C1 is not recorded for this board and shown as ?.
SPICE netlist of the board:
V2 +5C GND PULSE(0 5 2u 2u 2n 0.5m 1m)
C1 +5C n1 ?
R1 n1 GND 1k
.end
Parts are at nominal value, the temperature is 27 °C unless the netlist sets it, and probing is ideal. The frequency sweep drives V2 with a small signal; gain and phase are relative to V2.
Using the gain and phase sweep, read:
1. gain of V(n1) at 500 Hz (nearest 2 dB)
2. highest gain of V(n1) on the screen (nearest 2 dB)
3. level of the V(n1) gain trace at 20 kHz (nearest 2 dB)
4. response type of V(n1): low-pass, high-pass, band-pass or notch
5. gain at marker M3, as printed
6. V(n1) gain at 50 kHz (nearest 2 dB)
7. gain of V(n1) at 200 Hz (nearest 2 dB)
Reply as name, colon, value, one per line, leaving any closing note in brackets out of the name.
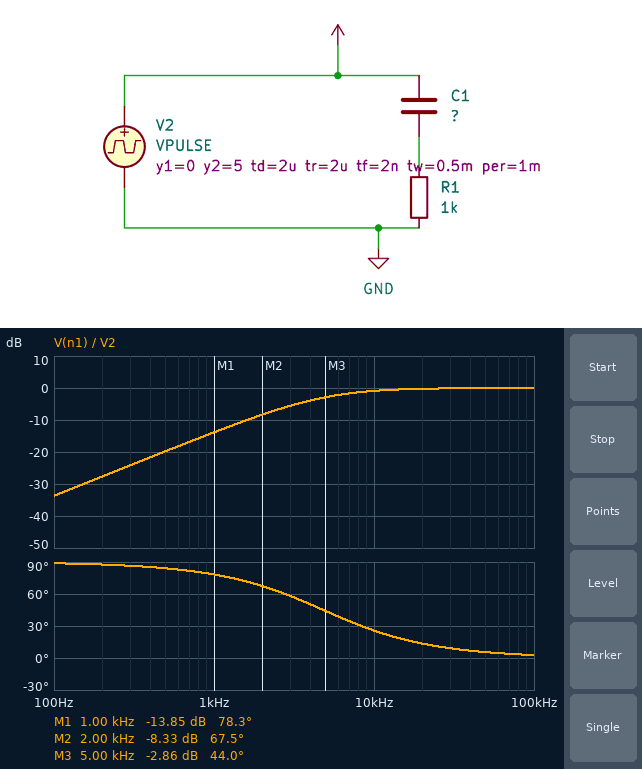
gain of V(n1) at 500 Hz: -20 dB
highest gain of V(n1) on the screen: 0 dB
level of the V(n1) gain trace at 20 kHz: 0 dB
response type of V(n1): low-pass, high-pass, band-pass or notch: high-pass
gain at marker M3, as printed: -2.86 dB
V(n1) gain at 50 kHz: 0 dB
gain of V(n1) at 200 Hz: -28 dB
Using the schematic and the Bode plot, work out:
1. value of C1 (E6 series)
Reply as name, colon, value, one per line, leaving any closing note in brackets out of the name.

value of C1: 33 nF
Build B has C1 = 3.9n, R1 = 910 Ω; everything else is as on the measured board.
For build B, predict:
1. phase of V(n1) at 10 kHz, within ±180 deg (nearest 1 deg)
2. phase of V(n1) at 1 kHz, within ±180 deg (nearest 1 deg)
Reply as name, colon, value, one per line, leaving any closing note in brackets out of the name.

phase of V(n1) at 10 kHz, within ±180 deg: 77 deg
phase of V(n1) at 1 kHz, within ±180 deg: 89 deg
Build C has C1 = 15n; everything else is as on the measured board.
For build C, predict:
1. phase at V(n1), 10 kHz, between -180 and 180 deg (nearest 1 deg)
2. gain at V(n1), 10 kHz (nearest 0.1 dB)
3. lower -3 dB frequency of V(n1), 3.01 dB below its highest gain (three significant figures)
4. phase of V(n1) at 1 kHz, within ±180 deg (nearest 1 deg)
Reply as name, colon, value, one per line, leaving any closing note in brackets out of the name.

phase at V(n1), 10 kHz, between -180 and 180 deg: 47 deg
gain at V(n1), 10 kHz: -3.3 dB
lower -3 dB frequency of V(n1), 3.01 dB below its highest gain: 10.6 kHz
phase of V(n1) at 1 kHz, within ±180 deg: 85 deg
